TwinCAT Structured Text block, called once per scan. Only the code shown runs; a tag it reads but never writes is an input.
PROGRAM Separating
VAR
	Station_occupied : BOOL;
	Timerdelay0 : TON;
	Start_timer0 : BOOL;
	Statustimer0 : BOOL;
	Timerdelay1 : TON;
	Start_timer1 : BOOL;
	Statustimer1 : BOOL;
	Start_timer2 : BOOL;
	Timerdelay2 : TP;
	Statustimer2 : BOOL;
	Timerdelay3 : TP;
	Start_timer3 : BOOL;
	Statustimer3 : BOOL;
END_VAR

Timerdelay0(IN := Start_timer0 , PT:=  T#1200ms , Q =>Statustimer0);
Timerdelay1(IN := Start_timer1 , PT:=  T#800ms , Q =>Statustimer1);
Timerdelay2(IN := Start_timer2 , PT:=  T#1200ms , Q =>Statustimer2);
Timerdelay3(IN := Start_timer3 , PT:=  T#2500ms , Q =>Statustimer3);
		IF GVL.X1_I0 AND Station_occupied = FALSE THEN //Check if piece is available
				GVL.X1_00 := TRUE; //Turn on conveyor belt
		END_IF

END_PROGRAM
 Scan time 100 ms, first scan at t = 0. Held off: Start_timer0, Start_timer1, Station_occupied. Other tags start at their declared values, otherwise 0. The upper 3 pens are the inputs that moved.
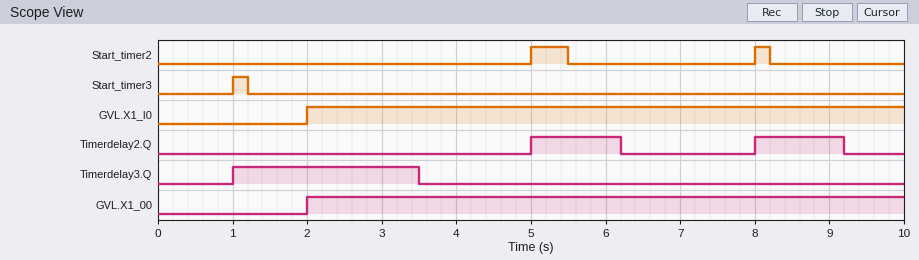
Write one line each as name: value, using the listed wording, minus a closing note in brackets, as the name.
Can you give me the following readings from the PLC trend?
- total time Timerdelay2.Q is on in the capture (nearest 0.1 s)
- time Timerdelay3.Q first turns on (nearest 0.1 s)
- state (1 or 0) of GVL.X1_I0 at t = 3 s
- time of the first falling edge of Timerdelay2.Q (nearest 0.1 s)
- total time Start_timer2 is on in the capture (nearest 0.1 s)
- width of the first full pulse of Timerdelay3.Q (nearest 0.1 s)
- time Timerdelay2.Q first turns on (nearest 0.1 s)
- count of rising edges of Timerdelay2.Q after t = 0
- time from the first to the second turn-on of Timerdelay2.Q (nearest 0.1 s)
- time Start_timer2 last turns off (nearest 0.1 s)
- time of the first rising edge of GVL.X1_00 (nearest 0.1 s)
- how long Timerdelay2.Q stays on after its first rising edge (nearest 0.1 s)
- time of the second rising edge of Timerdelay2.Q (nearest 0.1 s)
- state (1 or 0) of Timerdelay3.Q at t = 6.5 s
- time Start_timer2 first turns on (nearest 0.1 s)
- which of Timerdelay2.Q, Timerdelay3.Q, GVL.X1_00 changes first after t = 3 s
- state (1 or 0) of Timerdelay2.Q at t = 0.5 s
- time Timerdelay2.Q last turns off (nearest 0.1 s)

total time Timerdelay2.Q is on in the capture: 2.4 s
time Timerdelay3.Q first turns on: 1.0 s
state (1 or 0) of GVL.X1_I0 at t = 3 s: 1
time of the first falling edge of Timerdelay2.Q: 6.2 s
total time Start_timer2 is on in the capture: 0.7 s
width of the first full pulse of Timerdelay3.Q: 2.5 s
time Timerdelay2.Q first turns on: 5.0 s
count of rising edges of Timerdelay2.Q after t = 0: 2
time from the first to the second turn-on of Timerdelay2.Q: 3.0 s
time Start_timer2 last turns off: 8.2 s
time of the first rising edge of GVL.X1_00: 2.0 s
how long Timerdelay2.Q stays on after its first rising edge: 1.2 s
time of the second rising edge of Timerdelay2.Q: 8.0 s
state (1 or 0) of Timerdelay3.Q at t = 6.5 s: 0
time Start_timer2 first turns on: 5.0 s
which of Timerdelay2.Q, Timerdelay3.Q, GVL.X1_00 changes first after t = 3 s: Timerdelay3.Q
state (1 or 0) of Timerdelay2.Q at t = 0.5 s: 0
time Timerdelay2.Q last turns off: 9.2 s
